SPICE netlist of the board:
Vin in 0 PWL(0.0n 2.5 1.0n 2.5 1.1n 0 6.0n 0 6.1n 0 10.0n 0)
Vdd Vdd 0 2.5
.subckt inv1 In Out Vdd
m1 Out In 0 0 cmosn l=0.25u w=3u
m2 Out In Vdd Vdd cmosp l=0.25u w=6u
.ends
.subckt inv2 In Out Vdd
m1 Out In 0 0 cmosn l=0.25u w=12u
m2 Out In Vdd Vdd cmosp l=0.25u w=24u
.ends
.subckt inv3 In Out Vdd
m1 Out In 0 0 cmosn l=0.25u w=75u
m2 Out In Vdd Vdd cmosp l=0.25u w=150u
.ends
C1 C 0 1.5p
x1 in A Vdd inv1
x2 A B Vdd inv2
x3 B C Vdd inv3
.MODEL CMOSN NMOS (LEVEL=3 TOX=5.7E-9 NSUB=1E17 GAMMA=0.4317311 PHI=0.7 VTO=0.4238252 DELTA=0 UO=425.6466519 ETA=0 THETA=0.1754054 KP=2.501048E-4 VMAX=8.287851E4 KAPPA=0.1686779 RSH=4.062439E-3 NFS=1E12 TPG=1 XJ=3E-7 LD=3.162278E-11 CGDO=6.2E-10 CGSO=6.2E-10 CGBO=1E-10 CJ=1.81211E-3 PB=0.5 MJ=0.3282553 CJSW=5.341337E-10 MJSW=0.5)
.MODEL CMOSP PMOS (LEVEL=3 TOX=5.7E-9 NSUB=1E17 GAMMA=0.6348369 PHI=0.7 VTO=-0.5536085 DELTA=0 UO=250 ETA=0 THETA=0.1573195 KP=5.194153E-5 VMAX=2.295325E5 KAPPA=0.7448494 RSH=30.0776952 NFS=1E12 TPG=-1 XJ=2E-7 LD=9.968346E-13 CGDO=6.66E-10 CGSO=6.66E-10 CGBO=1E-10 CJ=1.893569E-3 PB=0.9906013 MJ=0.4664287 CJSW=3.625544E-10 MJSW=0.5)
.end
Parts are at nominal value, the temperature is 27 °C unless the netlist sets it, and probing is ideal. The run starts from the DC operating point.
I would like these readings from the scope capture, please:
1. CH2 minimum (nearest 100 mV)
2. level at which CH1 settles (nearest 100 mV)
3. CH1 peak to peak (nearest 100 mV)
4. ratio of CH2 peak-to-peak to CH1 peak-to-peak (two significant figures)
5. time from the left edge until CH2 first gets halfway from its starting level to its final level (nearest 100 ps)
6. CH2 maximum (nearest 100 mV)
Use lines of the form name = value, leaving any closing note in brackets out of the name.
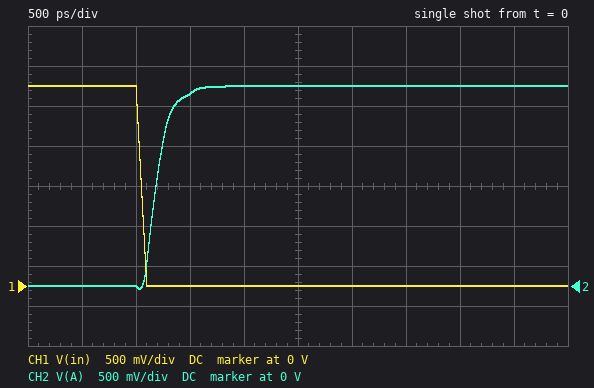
CH2 minimum = 0 V
level at which CH1 settles = 0 V
CH1 peak to peak = 2.5 V
ratio of CH2 peak-to-peak to CH1 peak-to-peak = 1.0
time from the left edge until CH2 first gets halfway from its starting level to its final level = 1.2 ns
CH2 maximum = 2.5 V
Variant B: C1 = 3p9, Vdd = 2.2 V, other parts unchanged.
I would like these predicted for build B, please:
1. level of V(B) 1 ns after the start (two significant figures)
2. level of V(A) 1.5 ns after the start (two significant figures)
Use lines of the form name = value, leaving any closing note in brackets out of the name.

level of V(B) 1 ns after the start = 2.2 V
level of V(A) 1.5 ns after the start = 2.1 V
